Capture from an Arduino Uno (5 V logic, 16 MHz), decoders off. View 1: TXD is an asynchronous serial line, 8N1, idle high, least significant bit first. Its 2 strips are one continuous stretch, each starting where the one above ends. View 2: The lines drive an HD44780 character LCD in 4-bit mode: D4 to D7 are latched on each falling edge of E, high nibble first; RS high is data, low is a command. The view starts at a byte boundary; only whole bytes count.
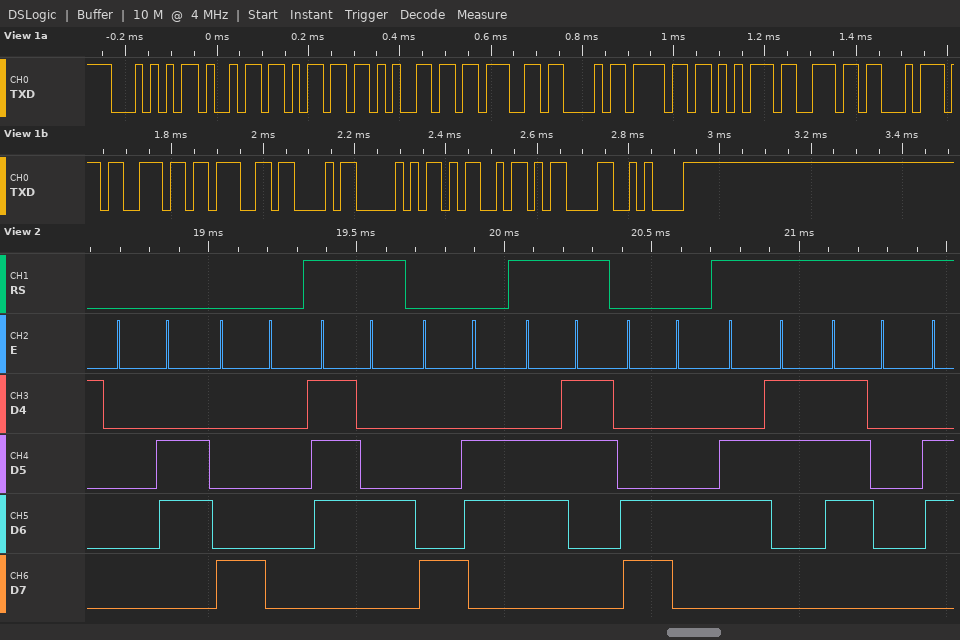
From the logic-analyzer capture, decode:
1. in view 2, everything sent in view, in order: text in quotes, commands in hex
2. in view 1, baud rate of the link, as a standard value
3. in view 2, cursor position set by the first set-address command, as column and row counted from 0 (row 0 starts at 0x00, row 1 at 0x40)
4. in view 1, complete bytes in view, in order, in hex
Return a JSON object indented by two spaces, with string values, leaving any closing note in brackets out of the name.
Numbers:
{
  "in view 2, everything sent in view, in order: text in quotes, commands in hex": "0x06 0x80 \"t\" 0x86 \"c\" 0xC4 \"cp\"",
  "in view 1, baud rate of the link, as a standard value": "57600 baud",
  "in view 2, cursor position set by the first set-address command, as column and row counted from 0": "column 0, row 0",
  "in view 1, complete bytes in view, in order, in hex": "0x54 0x69 0x6D 0x65 0x3B 0x43 0x6F 0x75 0x6E 0x74 0x73 0x3B 0x43 0x50 0x4D 0x0D 0x0A"
}
